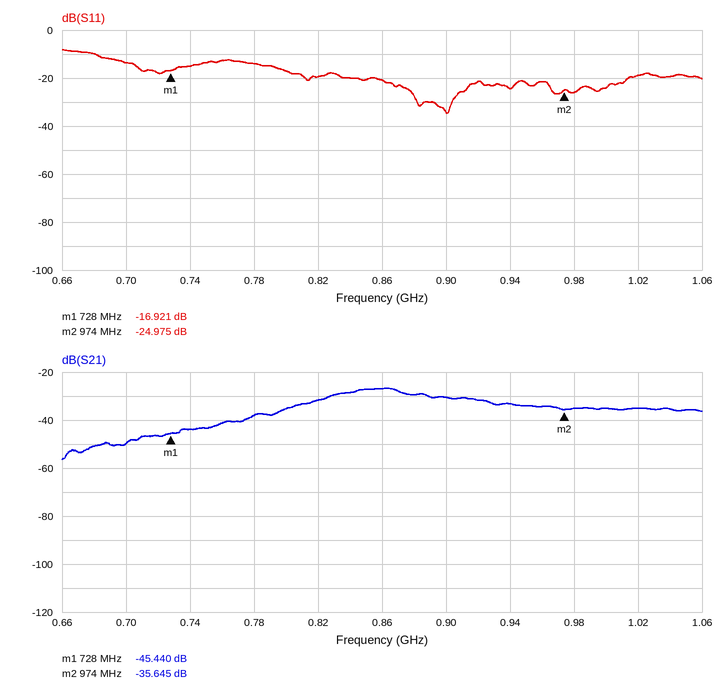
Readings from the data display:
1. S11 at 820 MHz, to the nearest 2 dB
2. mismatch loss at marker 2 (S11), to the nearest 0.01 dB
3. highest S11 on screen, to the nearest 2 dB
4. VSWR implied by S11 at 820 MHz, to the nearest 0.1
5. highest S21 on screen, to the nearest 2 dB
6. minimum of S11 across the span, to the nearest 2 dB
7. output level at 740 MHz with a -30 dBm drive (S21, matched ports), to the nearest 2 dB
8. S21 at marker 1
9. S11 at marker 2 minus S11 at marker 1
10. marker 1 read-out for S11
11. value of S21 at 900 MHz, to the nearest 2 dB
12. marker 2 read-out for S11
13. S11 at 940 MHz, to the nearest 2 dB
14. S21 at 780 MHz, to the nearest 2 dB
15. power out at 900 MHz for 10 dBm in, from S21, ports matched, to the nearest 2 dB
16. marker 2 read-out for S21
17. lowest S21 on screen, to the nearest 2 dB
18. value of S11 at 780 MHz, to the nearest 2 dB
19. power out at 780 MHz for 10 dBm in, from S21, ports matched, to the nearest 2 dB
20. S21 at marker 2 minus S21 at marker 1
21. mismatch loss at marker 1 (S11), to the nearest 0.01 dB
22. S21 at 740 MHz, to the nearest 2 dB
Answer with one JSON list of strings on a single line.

["-20 dB", "0.01 dB", "-8 dB", "1.2", "-26 dB", "-34 dB", "-74 dBm", "-45.440 dB", "-8.054 dB", "-16.921 dB", "-30 dB", "-24.975 dB", "-24 dB", "-38 dB", "-20 dBm", "-35.645 dB", "-56 dB", "-14 dB", "-28 dBm", "9.795 dB", "0.09 dB", "-44 dB"]
